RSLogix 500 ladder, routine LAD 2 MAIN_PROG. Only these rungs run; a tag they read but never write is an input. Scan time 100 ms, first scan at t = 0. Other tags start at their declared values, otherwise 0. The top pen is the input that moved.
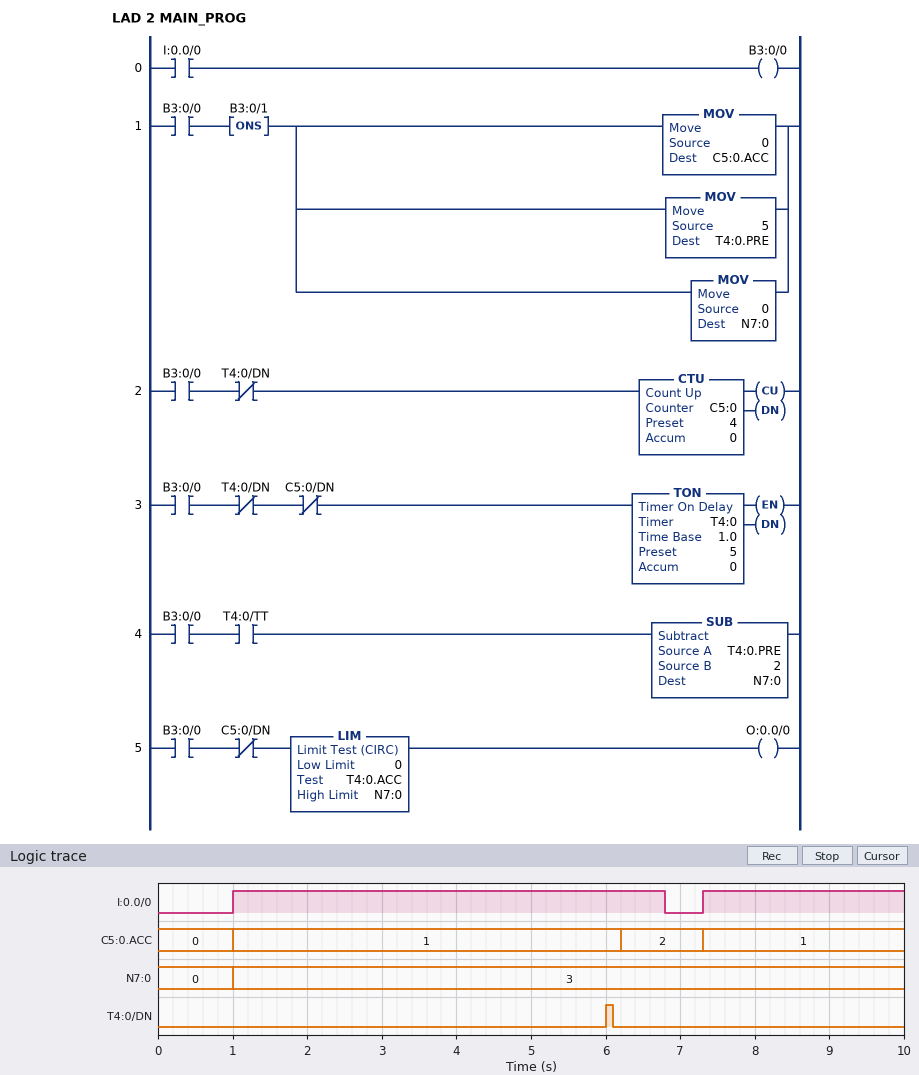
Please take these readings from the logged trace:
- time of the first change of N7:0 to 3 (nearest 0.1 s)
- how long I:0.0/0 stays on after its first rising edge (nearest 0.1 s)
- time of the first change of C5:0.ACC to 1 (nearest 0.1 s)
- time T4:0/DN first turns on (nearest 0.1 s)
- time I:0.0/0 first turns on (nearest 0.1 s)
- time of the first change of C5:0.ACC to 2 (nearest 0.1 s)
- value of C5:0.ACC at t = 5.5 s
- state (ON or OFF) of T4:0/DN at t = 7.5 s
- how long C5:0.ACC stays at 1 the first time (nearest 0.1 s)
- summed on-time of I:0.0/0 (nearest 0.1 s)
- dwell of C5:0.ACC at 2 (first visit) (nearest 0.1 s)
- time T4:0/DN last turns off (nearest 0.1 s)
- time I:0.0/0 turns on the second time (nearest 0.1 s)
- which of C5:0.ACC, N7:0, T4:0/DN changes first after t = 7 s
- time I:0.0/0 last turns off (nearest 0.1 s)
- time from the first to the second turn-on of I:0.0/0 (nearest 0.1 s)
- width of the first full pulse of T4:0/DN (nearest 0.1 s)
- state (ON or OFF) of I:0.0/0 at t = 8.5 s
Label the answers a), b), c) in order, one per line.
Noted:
a) 1.0 s
b) 5.8 s
c) 1.0 s
d) 6.0 s
e) 1.0 s
f) 6.2 s
g) 1
h) OFF
i) 5.2 s
j) 8.5 s
k) 1.1 s
l) 6.1 s
m) 7.3 s
n) C5:0.ACC
o) 6.8 s
p) 6.3 s
q) 0.1 s
r) ON
